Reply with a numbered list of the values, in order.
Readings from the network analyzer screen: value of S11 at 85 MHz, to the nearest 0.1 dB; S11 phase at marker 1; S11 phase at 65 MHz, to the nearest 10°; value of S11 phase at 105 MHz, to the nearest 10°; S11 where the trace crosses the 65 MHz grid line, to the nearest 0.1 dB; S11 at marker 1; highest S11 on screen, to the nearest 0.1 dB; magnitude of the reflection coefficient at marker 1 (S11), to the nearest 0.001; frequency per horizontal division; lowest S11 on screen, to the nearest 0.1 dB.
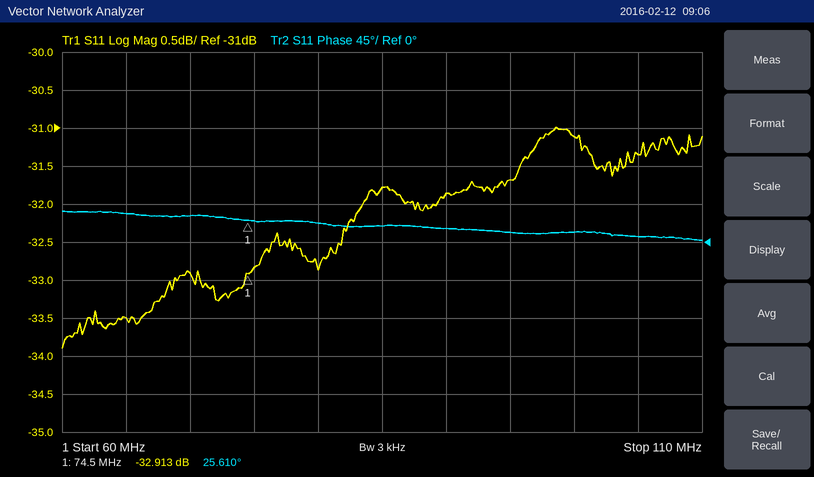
1. -31.8 dB
2. 25.610°
3. 30°
4. 10°
5. -33.5 dB
6. -32.913 dB
7. -31.0 dB
8. 0.023
9. 5 MHz
10. -33.9 dB
